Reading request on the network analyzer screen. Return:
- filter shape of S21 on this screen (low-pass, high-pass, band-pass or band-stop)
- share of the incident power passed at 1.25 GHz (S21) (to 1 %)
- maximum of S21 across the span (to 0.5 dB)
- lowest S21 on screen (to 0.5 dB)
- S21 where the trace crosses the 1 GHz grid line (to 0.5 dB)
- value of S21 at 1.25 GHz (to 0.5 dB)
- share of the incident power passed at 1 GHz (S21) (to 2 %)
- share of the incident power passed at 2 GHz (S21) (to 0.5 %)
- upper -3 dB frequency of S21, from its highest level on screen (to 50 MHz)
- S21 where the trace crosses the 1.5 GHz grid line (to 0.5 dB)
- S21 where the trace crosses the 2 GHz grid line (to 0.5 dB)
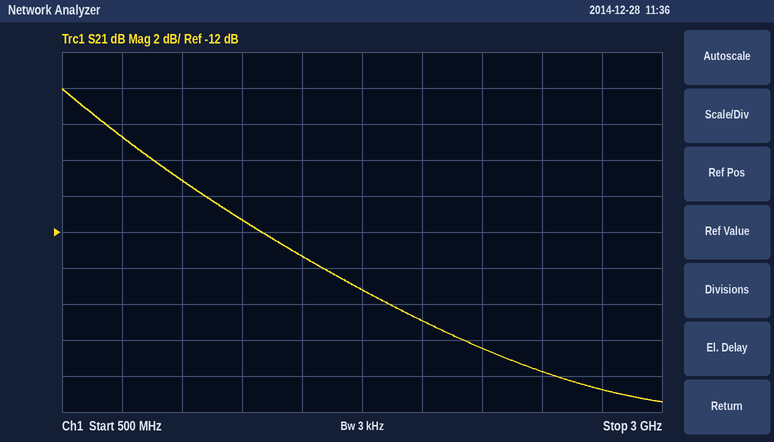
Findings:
low-pass
7 %
-4.0 dB
-21.5 dB
-9.0 dB
-11.5 dB
12 %
2.0 %
800 MHz
-13.5 dB
-17.0 dB
